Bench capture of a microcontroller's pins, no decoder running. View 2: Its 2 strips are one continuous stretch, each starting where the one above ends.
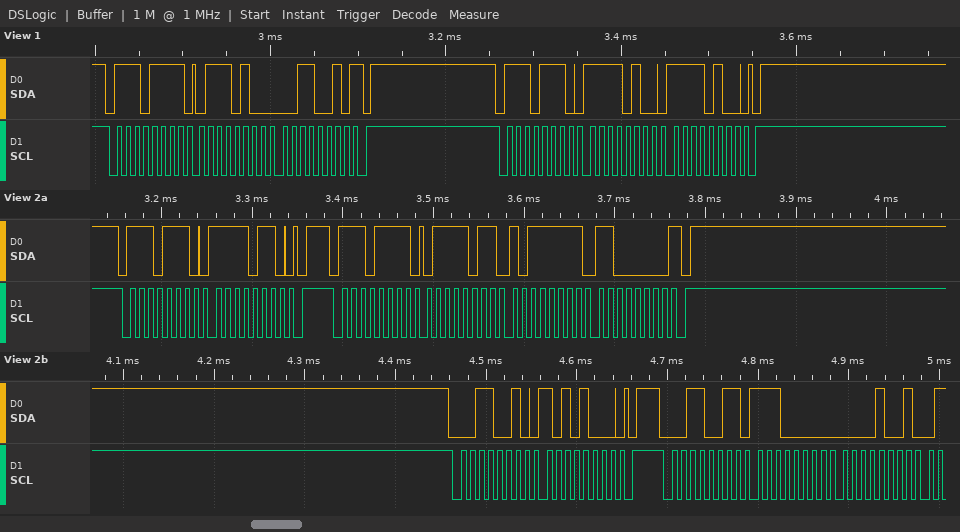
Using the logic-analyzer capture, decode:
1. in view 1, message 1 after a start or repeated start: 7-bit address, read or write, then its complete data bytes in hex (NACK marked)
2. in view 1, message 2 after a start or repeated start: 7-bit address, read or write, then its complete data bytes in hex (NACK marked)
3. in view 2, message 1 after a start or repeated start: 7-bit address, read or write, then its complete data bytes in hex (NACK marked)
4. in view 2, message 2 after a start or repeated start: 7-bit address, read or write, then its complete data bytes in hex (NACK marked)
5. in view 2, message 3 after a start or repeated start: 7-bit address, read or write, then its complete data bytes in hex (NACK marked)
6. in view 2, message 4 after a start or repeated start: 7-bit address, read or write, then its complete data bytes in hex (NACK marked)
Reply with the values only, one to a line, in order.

0x77 read: 74 32 NACK
0x77 write: F4 F4
0x77 write: F6
0x77 read: 7B BF C0 NACK
0x19 write: A8
0x19 read: E0 09
